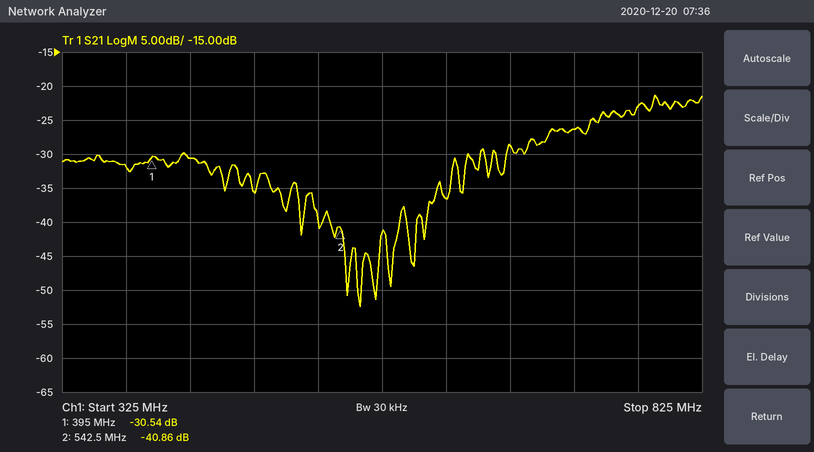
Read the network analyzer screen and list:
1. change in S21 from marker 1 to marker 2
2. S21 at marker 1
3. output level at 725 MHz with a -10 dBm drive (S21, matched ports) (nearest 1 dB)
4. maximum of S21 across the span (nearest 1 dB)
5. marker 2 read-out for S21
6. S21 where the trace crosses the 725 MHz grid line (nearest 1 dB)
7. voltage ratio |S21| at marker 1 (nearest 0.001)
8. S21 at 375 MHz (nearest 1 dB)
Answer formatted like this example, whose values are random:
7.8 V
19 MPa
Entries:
-10.32 dB
-30.54 dB
-36 dBm
-21 dB
-40.86 dB
-26 dB
0.030
-32 dB
